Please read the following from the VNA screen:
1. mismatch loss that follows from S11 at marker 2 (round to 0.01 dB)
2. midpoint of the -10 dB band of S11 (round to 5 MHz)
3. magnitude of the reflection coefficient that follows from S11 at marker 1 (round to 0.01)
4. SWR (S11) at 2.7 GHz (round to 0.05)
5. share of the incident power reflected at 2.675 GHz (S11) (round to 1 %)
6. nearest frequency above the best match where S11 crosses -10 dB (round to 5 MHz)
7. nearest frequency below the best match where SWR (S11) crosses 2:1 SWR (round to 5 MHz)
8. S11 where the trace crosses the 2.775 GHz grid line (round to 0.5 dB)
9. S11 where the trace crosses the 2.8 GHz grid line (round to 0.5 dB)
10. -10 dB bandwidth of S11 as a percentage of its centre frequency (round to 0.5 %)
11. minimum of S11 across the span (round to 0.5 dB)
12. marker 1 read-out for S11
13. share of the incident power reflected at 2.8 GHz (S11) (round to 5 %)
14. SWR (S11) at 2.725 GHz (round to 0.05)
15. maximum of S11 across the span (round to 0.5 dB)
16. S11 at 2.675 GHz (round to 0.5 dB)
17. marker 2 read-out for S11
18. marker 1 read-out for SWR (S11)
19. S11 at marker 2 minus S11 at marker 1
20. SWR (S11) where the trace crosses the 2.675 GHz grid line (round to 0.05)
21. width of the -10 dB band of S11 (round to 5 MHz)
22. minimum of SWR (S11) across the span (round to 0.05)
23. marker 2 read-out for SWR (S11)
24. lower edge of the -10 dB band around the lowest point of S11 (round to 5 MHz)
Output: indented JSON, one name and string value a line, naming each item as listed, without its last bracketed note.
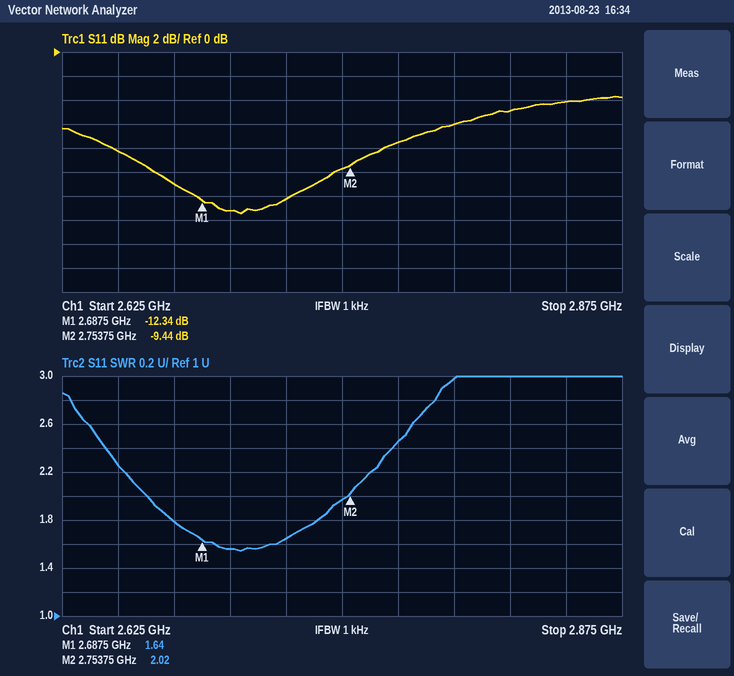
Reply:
{
  "mismatch loss that follows from S11 at marker 2": "0.52 dB",
  "midpoint of the -10 dB band of S11": "2.705 GHz",
  "magnitude of the reflection coefficient that follows from S11 at marker 1": "0.24",
  "SWR (S11) at 2.7 GHz": "1.55",
  "share of the incident power reflected at 2.675 GHz (S11)": "8 %",
  "nearest frequency above the best match where S11 crosses -10 dB": "2.745 GHz",
  "nearest frequency below the best match where SWR (S11) crosses 2:1 SWR": "2.665 GHz",
  "S11 where the trace crosses the 2.775 GHz grid line": "-7.5 dB",
  "S11 where the trace crosses the 2.8 GHz grid line": "-6.0 dB",
  "-10 dB bandwidth of S11 as a percentage of its centre frequency": "3.0 %",
  "minimum of S11 across the span": "-13.5 dB",
  "marker 1 read-out for S11": "-12.34 dB",
  "share of the incident power reflected at 2.8 GHz (S11)": "25 %",
  "SWR (S11) at 2.725 GHz": "1.65",
  "maximum of S11 across the span": "-3.5 dB",
  "S11 at 2.675 GHz": "-11.0 dB",
  "marker 2 read-out for S11": "-9.44 dB",
  "marker 1 read-out for SWR": "1.64",
  "S11 at marker 2 minus S11 at marker 1": "2.90 dB",
  "SWR (S11) where the trace crosses the 2.675 GHz grid line": "1.80",
  "width of the -10 dB band of S11": "80 MHz",
  "minimum of SWR (S11) across the span": "1.55",
  "marker 2 read-out for SWR": "2.02",
  "lower edge of the -10 dB band around the lowest point of S11": "2.665 GHz"
}
